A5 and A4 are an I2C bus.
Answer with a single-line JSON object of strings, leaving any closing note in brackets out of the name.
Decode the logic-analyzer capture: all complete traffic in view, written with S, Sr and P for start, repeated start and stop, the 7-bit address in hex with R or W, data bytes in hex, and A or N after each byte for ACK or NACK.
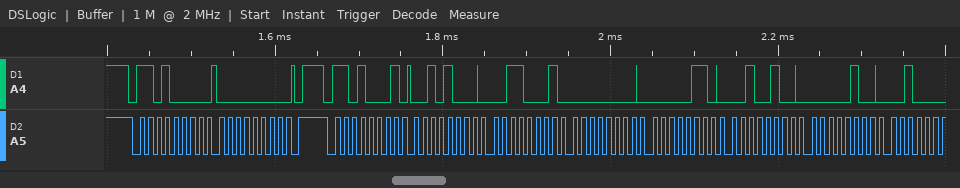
{"all complete traffic in view, written with S, Sr and P for start, repeated start and stop, the 7-bit address in hex with R or W, data bytes in hex, and A or N after each byte for ACK or NACK": "S 68W A 00 A P S 68R A 28 A 31 A 00 A 06 A 24 A 04 A"}
